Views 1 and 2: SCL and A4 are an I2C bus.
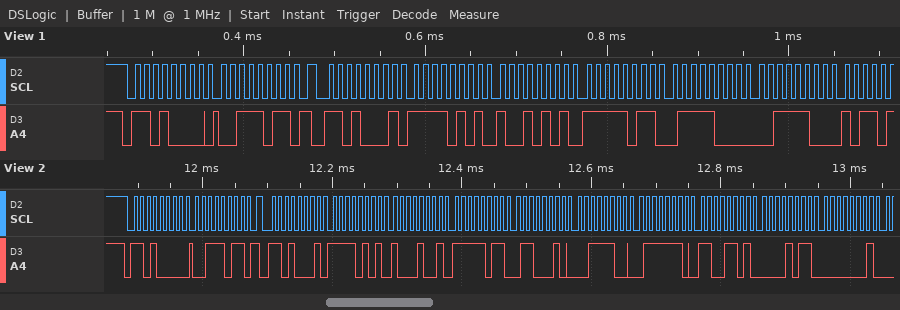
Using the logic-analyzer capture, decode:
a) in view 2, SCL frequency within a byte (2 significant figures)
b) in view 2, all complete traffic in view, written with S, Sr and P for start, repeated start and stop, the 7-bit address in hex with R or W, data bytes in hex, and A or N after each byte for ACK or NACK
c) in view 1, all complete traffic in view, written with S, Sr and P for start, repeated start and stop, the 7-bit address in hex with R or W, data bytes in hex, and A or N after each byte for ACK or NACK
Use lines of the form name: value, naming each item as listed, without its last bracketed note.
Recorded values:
in view 2, SCL frequency within a byte: 100 kHz
in view 2, all complete traffic in view, written with S, Sr and P for start, repeated start and stop, the 7-bit address in hex with R or W, data bytes in hex, and A or N after each byte for ACK or NACK: S 68W A 3B A Sr 68R A F5 A 89 A FB A 62 A 3C A 7E A CD A 0B A 01 A
in view 1, all complete traffic in view, written with S, Sr and P for start, repeated start and stop, the 7-bit address in hex with R or W, data bytes in hex, and A or N after each byte for ACK or NACK: S 68W A 3B A Sr 68R A F5 A 95 A FB A 78 A 3C A
